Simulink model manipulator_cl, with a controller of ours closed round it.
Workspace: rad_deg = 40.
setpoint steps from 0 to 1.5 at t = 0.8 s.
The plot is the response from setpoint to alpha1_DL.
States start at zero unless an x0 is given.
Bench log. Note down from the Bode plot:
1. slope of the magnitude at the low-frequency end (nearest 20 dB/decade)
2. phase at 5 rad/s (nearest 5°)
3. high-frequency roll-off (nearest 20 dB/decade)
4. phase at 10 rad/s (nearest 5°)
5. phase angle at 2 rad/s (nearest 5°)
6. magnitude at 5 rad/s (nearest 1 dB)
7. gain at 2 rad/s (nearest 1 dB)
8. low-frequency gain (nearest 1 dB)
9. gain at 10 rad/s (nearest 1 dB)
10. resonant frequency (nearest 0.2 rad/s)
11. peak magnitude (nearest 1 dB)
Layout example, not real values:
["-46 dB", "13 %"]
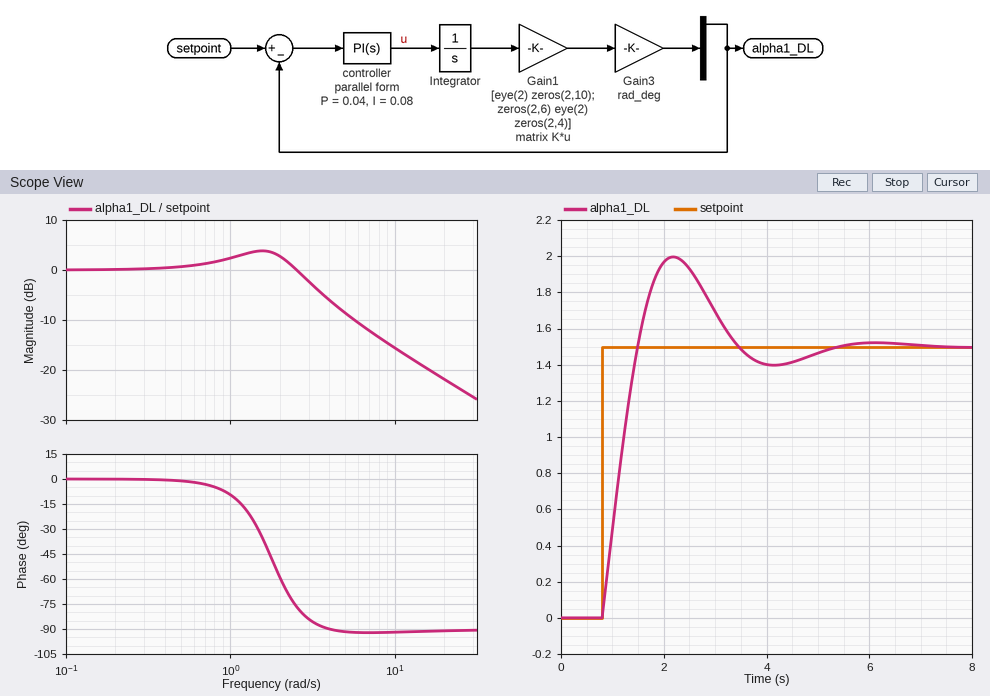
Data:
["0 dB/decade", "-90°", "-20 dB/decade", "-90°", "-60°", "-9 dB", "3 dB", "0 dB", "-16 dB", "1.6 rad/s", "4 dB"]
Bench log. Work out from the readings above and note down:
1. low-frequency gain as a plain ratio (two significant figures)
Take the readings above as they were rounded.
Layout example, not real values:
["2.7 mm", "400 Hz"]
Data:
["1.0"]
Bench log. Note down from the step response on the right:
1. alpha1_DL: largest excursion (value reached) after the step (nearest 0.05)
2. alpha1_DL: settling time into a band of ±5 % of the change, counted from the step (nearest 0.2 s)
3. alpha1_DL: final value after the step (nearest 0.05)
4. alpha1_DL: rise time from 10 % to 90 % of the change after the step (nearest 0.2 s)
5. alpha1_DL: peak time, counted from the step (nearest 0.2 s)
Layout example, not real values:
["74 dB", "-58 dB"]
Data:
["2.00", "3.8 s", "1.50", "0.6 s", "1.4 s"]
